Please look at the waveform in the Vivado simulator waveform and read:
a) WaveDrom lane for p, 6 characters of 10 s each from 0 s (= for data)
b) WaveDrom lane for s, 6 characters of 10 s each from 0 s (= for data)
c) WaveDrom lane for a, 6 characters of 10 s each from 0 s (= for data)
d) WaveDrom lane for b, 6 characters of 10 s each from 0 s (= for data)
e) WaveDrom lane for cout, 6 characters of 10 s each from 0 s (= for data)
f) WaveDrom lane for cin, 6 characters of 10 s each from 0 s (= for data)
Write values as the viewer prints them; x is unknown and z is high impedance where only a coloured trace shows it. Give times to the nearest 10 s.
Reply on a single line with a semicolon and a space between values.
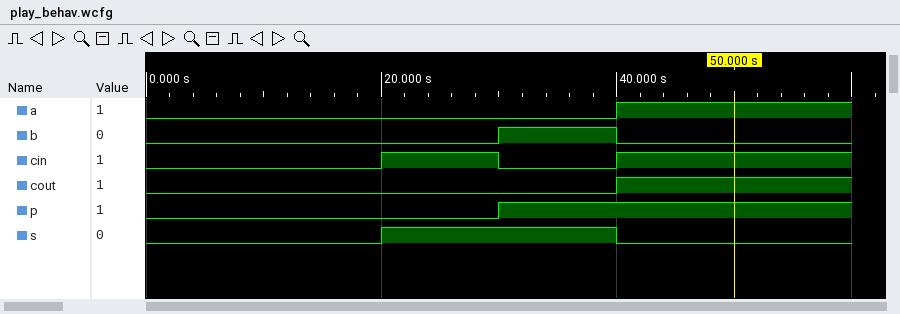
{name: 'p', wave: '0..1..'}; {name: 's', wave: '0.1.0.'}; {name: 'a', wave: '0...1.'}; {name: 'b', wave: '0..10.'}; {name: 'cout', wave: '0...1.'}; {name: 'cin', wave: '0.101.'}
